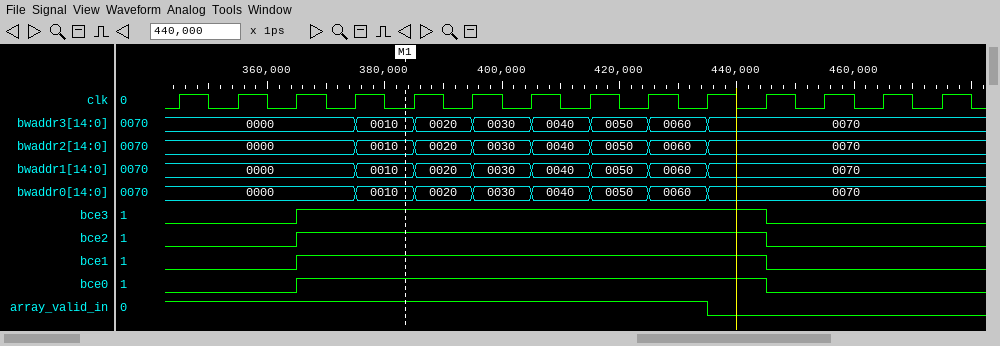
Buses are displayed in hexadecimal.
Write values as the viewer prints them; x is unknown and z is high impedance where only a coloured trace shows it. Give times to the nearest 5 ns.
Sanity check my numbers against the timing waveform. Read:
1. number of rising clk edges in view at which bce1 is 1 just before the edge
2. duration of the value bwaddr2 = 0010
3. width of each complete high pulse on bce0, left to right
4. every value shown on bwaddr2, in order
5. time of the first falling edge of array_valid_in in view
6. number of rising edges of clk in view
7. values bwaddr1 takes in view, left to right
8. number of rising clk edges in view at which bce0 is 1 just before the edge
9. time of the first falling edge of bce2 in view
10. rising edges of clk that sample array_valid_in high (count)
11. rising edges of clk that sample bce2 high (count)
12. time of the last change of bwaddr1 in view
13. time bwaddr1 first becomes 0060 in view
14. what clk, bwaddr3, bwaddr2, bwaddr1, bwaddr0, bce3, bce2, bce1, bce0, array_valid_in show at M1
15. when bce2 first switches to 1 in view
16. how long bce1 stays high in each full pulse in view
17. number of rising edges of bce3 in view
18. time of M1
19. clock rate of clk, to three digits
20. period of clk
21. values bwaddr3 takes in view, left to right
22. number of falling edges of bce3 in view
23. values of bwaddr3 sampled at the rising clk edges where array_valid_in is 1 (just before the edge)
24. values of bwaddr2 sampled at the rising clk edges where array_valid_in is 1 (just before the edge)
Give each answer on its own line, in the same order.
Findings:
8
10 ns
80 ns
0000, 0010, 0020, 0030, 0040, 0050, 0060, 0070
435 ns
14
0000, 0010, 0020, 0030, 0040, 0050, 0060, 0070
8
445 ns
10
8
435 ns
425 ns
clk=0, bwaddr3=0010, bwaddr2=0010, bwaddr1=0010, bwaddr0=0010, bce3=1, bce2=1, bce1=1, bce0=1, array_valid_in=1
365 ns
80 ns
1
385 ns
100 MHz
10 ns
0000, 0010, 0020, 0030, 0040, 0050, 0060, 0070
1
0000, 0000, 0000, 0000, 0010, 0020, 0030, 0040, 0050, 0060
0000, 0000, 0000, 0000, 0010, 0020, 0030, 0040, 0050, 0060
